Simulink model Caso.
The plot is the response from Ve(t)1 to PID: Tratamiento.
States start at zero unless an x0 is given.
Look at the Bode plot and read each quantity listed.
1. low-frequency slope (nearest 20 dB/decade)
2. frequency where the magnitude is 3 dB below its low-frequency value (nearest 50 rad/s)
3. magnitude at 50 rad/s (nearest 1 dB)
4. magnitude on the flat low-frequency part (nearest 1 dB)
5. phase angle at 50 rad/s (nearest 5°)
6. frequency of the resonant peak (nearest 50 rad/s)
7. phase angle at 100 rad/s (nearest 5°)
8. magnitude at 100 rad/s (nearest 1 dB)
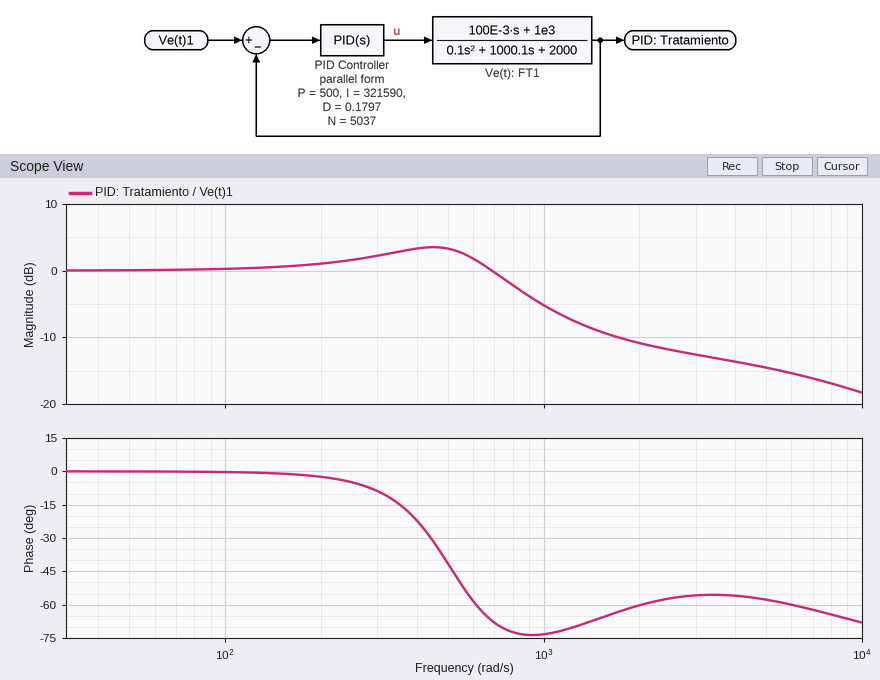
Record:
0 dB/decade
850 rad/s
0 dB
0 dB
0°
450 rad/s
0°
0 dB
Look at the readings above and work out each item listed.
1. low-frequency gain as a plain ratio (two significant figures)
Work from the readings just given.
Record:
1.0
